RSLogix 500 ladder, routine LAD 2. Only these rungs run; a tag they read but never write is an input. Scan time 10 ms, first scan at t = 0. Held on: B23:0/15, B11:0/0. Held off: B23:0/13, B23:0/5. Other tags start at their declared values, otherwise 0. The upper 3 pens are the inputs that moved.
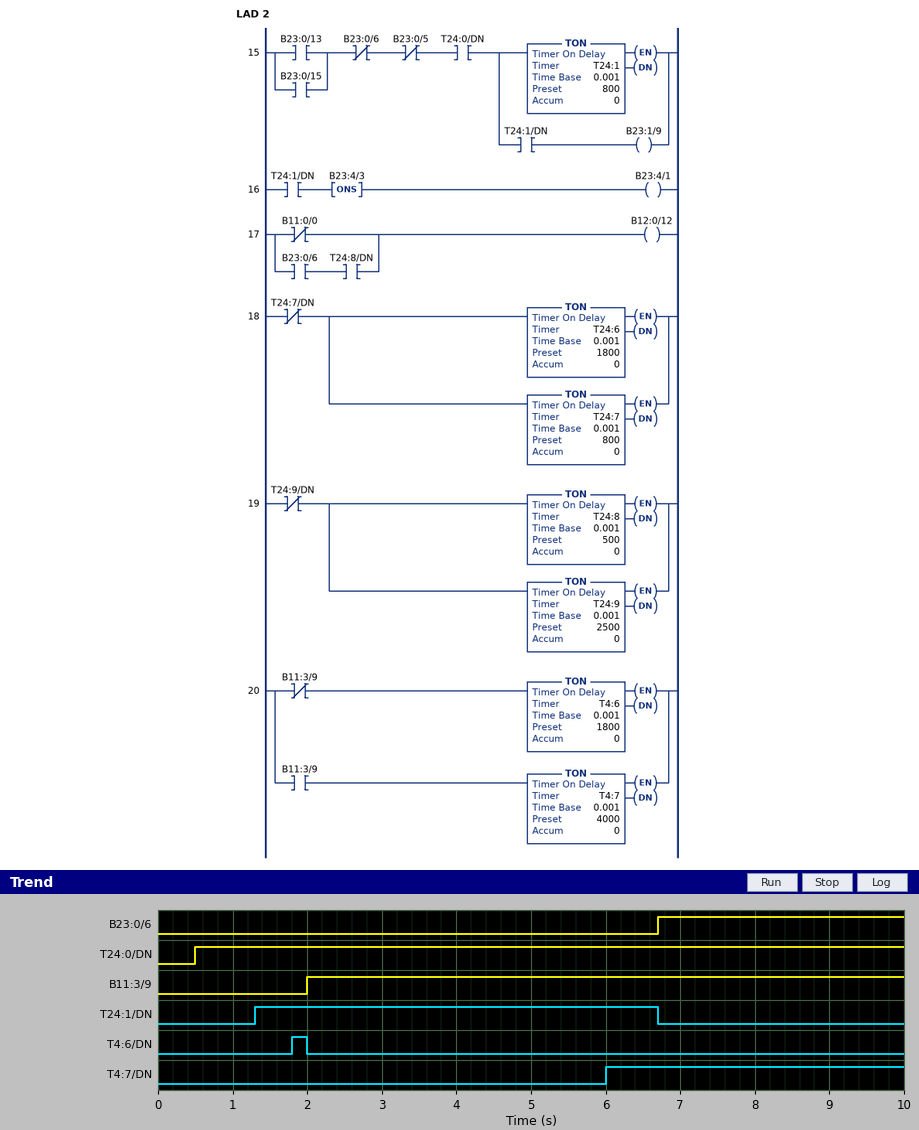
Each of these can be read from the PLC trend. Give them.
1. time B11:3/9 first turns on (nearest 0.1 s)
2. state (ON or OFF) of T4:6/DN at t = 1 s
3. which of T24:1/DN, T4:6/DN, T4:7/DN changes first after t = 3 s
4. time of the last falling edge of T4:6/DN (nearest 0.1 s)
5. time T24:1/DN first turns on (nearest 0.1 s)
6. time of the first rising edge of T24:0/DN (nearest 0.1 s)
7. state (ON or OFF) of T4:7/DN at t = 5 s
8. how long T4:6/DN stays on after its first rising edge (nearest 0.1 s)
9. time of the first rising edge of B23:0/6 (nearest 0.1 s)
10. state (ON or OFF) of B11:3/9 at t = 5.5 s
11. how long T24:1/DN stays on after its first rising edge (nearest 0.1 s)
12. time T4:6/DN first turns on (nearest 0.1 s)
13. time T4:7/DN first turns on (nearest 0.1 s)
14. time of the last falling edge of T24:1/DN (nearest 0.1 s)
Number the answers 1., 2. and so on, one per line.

1. 2.0 s
2. OFF
3. T4:7/DN
4. 2.0 s
5. 1.3 s
6. 0.5 s
7. OFF
8. 0.2 s
9. 6.7 s
10. ON
11. 5.4 s
12. 1.8 s
13. 6.0 s
14. 6.7 s
